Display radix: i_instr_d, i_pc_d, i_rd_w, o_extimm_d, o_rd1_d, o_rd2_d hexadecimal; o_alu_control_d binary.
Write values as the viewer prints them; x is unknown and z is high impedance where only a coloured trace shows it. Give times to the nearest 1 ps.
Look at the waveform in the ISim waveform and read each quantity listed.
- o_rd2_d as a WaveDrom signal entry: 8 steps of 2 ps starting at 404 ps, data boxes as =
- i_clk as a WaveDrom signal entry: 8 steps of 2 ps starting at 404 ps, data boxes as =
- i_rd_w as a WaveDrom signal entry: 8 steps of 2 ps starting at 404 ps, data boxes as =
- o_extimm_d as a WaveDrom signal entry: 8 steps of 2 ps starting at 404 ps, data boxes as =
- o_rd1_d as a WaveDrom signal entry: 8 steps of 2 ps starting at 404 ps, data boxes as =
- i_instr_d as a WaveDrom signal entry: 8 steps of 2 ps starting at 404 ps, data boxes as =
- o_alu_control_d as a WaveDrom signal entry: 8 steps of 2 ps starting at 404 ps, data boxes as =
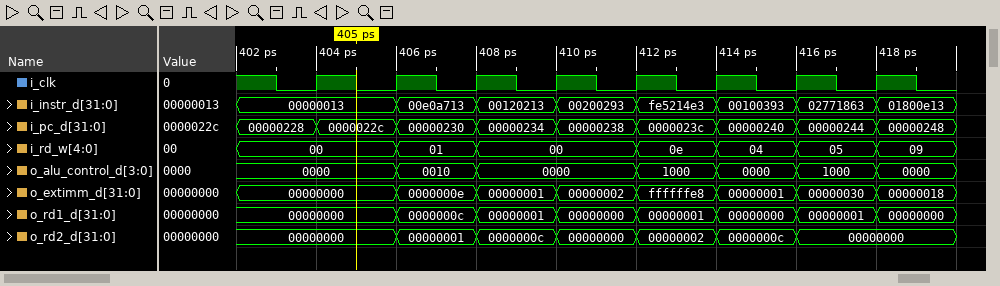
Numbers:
{name: 'o_rd2_d', wave: '=======.', data: '00000000 00000001 0000000c 00000000 00000002 0000000c 00000000'}
{name: 'i_clk', wave: 'p.......'}
{name: 'i_rd_w', wave: '===.====', data: '00 01 00 0e 04 05 09'}
{name: 'o_extimm_d', wave: '========', data: '00000000 0000000e 00000001 00000002 ffffffe8 00000001 00000030 00000018'}
{name: 'o_rd1_d', wave: '========', data: '00000000 0000000c 00000001 00000000 00000001 00000000 00000001 00000000'}
{name: 'i_instr_d', wave: '========', data: '00000013 00e0a713 00120213 00200293 fe5214e3 00100393 02771863 01800e13'}
{name: 'o_alu_control_d', wave: '===.====', data: '0000 0010 0000 1000 0000 1000 0000'}
